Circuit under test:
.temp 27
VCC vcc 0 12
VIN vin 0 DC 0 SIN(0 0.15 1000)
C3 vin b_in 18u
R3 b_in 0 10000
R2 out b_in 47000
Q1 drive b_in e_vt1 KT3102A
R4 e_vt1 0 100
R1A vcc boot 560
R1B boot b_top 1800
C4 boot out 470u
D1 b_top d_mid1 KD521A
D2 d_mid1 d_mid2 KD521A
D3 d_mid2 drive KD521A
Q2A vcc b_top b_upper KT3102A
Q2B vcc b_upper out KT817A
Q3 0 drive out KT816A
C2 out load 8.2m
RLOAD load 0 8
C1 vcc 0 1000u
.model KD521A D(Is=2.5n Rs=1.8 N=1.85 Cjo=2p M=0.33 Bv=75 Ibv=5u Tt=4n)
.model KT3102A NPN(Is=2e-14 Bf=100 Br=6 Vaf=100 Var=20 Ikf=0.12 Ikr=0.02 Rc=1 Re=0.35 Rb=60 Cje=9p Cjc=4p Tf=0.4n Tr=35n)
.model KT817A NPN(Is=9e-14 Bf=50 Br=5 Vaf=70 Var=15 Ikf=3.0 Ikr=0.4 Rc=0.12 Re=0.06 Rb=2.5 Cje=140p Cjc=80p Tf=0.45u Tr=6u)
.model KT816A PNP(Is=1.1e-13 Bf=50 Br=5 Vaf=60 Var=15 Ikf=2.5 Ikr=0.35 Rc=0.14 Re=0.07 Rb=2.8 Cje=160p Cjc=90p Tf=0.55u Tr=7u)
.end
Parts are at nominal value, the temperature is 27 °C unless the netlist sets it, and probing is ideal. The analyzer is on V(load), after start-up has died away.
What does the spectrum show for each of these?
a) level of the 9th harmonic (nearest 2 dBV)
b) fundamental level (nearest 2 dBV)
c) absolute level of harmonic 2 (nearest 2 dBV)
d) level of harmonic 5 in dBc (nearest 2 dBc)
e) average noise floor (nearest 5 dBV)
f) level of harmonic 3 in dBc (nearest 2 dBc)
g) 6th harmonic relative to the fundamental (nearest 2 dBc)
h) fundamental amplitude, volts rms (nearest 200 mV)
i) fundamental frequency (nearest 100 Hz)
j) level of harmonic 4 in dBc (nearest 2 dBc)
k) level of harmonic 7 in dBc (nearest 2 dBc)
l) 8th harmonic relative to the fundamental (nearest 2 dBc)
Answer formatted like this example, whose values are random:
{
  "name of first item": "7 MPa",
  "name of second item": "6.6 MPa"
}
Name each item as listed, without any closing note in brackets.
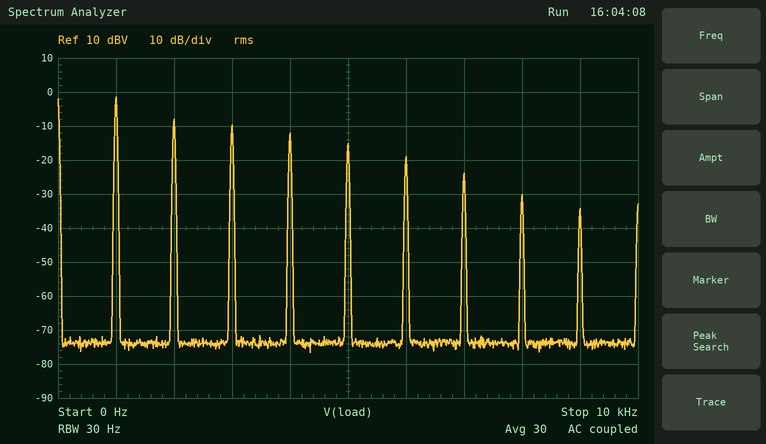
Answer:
{
  "level of the 9th harmonic": "-34 dBV",
  "fundamental level": "-2 dBV",
  "absolute level of harmonic 2": "-8 dBV",
  "level of harmonic 5 in dBc": "-14 dBc",
  "average noise floor": "-75 dBV",
  "level of harmonic 3 in dBc": "-8 dBc",
  "6th harmonic relative to the fundamental": "-18 dBc",
  "fundamental amplitude, volts rms": "800 mV",
  "fundamental frequency": "1.0 kHz",
  "level of harmonic 4 in dBc": "-10 dBc",
  "level of harmonic 7 in dBc": "-22 dBc",
  "8th harmonic relative to the fundamental": "-28 dBc"
}
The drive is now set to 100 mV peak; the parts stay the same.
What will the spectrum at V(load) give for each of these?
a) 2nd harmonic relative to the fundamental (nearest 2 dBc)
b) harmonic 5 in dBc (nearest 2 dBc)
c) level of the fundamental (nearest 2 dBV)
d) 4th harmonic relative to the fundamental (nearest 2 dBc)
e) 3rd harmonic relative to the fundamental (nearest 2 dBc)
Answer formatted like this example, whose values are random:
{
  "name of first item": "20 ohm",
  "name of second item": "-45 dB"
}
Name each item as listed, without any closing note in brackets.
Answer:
{
  "2nd harmonic relative to the fundamental": "-8 dBc",
  "harmonic 5 in dBc": "-16 dBc",
  "level of the fundamental": "-6 dBV",
  "4th harmonic relative to the fundamental": "-12 dBc",
  "3rd harmonic relative to the fundamental": "-10 dBc"
}
